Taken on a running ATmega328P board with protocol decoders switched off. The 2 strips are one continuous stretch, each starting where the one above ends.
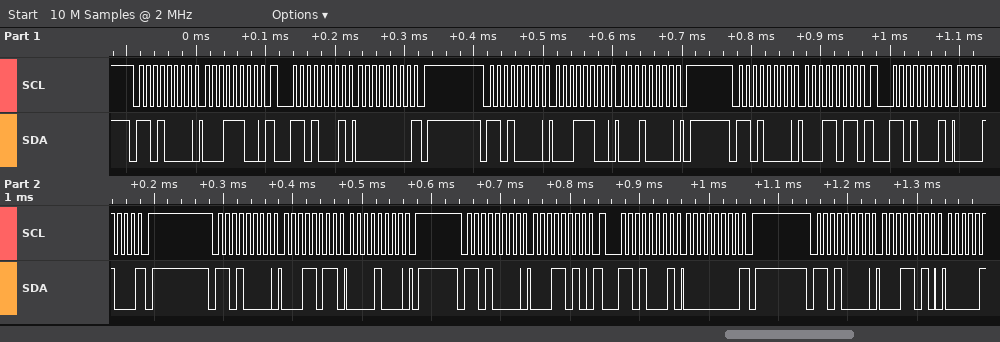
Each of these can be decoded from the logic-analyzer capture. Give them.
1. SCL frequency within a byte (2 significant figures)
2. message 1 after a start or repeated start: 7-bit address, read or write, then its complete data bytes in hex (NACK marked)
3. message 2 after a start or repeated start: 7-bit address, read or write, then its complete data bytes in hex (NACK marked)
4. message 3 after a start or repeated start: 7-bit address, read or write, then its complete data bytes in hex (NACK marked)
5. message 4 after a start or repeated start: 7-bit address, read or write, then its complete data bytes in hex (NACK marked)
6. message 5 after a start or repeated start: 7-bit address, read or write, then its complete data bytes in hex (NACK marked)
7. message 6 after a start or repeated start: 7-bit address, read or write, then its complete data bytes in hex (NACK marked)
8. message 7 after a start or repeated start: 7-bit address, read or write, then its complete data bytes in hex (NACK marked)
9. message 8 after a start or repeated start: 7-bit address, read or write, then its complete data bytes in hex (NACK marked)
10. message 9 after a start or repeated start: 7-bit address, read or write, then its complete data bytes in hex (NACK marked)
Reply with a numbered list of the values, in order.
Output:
1. 100 kHz
2. 0x68 write: 1C
3. 0x68 read: 00 NACK
4. 0x68 write: 1C 10
5. 0x68 write: 1B
6. 0x68 read: 08 NACK
7. 0x68 write: 1B 08
8. 0x68 write: 1A
9. 0x68 read: 00 NACK
10. 0x68 write: 1A
